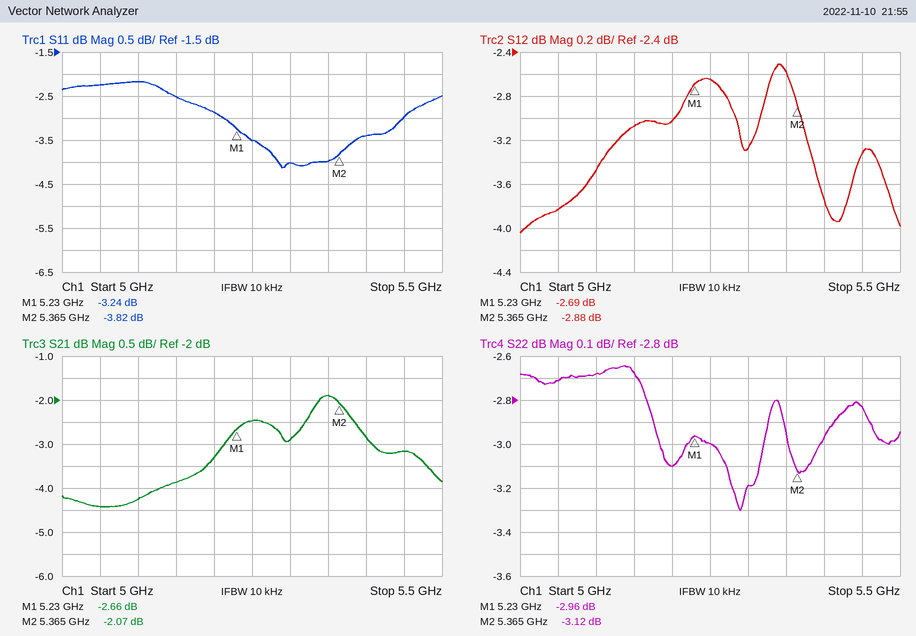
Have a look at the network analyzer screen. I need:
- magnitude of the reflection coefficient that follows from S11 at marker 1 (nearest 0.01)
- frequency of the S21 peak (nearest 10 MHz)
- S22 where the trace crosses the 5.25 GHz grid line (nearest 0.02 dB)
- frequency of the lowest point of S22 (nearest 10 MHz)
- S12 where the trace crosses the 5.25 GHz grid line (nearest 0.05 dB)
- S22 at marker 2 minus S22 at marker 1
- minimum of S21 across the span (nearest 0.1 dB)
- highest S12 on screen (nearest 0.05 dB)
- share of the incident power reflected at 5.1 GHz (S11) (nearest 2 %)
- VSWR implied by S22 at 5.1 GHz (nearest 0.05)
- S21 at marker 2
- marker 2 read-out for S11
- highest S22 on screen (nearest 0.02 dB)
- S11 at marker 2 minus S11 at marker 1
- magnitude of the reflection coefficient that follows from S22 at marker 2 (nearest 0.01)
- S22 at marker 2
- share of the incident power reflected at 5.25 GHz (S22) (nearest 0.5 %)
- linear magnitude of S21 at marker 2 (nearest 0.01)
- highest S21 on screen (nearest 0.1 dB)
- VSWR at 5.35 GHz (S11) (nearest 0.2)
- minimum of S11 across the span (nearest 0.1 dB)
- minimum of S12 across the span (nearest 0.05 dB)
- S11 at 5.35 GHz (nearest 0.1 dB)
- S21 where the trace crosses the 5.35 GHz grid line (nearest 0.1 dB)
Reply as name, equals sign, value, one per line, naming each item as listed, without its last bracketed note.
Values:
magnitude of the reflection coefficient that follows from S11 at marker 1 = 0.69
frequency of the S21 peak = 5.35 GHz
S22 where the trace crosses the 5.25 GHz grid line = -3.00 dB
frequency of the lowest point of S22 = 5.29 GHz
S12 where the trace crosses the 5.25 GHz grid line = -2.65 dB
S22 at marker 2 minus S22 at marker 1 = -0.16 dB
minimum of S21 across the span = -4.4 dB
highest S12 on screen = -2.50 dB
share of the incident power reflected at 5.1 GHz (S11) = 60 %
VSWR implied by S22 at 5.1 GHz = 6.55
S21 at marker 2 = -2.07 dB
marker 2 read-out for S11 = -3.82 dB
highest S22 on screen = -2.64 dB
S11 at marker 2 minus S11 at marker 1 = -0.58 dB
magnitude of the reflection coefficient that follows from S22 at marker 2 = 0.70
S22 at marker 2 = -3.12 dB
share of the incident power reflected at 5.25 GHz (S22) = 50.0 %
linear magnitude of S21 at marker 2 = 0.79
highest S21 on screen = -1.9 dB
VSWR at 5.35 GHz (S11) = 4.4
minimum of S11 across the span = -4.1 dB
minimum of S12 across the span = -4.05 dB
S11 at 5.35 GHz = -4.0 dB
S21 where the trace crosses the 5.35 GHz grid line = -1.9 dB
